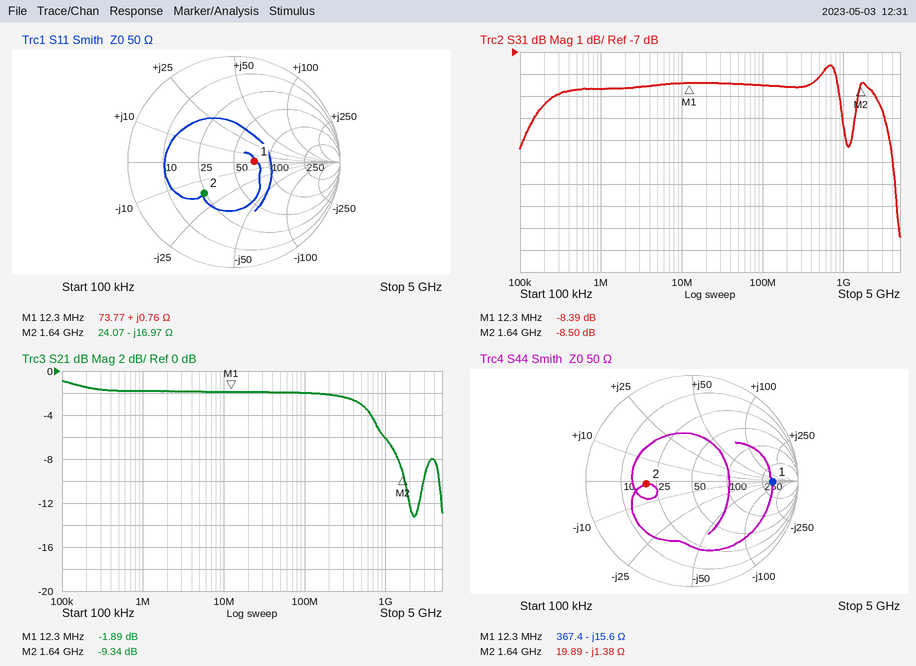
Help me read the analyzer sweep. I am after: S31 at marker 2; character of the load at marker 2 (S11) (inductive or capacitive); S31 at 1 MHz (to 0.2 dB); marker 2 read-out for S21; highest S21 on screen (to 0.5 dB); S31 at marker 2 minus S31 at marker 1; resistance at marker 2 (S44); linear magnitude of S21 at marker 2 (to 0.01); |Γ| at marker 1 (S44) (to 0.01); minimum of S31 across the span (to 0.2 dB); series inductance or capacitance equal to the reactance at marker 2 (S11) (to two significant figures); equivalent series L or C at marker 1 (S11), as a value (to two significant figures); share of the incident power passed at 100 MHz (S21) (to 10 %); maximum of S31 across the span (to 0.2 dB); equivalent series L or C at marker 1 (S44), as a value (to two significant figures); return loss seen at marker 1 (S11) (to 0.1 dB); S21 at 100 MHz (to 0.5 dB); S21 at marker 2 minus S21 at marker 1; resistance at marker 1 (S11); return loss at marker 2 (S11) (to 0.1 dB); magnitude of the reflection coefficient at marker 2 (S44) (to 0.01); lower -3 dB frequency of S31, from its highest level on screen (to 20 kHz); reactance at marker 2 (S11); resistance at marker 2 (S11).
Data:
-8.50 dB
capacitive
-8.6 dB
-9.34 dB
-1.0 dB
-0.11 dB
19.89 Ω
0.34
0.76
-15.4 dB
5.7 pF
9.8 nH
60 %
-7.6 dB
830 pF
14.3 dB
-2.0 dB
-7.45 dB
73.77 Ω
7.8 dB
0.43
120 kHz
-16.97 Ω
24.07 Ω
